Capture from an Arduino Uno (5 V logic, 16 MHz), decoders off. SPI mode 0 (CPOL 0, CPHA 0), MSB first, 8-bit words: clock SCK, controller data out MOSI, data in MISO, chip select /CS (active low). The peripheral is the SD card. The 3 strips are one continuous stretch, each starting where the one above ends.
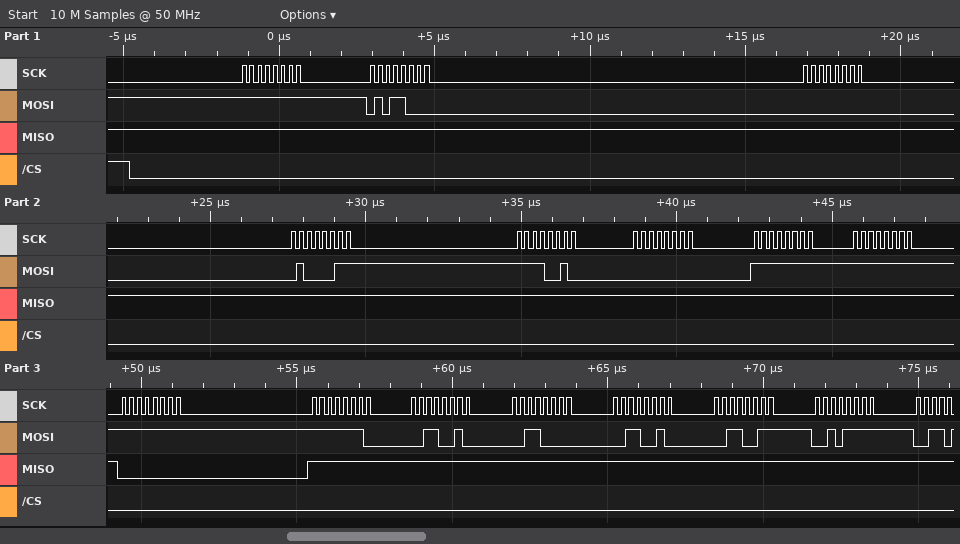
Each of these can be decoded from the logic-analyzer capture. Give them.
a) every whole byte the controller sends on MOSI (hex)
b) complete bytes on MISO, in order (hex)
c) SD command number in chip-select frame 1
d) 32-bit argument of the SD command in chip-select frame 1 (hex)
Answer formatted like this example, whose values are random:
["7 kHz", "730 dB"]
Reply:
["0xFF 0x58 0x00 0x43 0xF2 0x00 0xFF 0xFF 0xFF 0xFE 0x32 0x30 0x32 0x33 0x2F", "0xFF 0xFF 0xFF 0xFF 0xFF 0xFF 0xFF 0xFF 0x00 0xFF 0xFF 0xFF 0xFF 0xFF 0xFF", "CMD24", "0x0043F200"]
